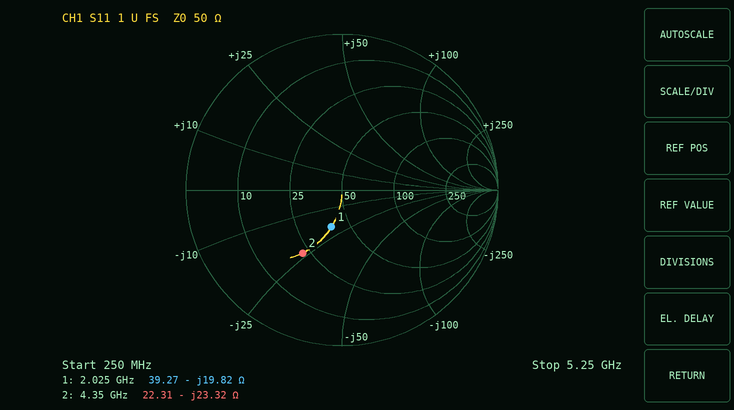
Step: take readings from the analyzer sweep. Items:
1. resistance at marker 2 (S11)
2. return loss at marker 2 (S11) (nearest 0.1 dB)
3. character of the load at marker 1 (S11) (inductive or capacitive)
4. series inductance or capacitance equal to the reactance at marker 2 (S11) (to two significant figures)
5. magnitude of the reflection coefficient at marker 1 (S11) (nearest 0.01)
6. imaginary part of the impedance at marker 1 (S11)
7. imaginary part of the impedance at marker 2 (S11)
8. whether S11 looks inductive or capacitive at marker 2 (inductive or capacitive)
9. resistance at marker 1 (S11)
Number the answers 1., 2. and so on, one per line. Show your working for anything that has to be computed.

1. 22.31 Ω
2. 6.4 dB
3. capacitive
4. C = 1/(2π × 4.35 GHz × 23.32 Ω) ≈ 1.6 pF
5. 0.25
6. -19.82 Ω
7. -23.32 Ω
8. capacitive
9. 39.27 Ω
